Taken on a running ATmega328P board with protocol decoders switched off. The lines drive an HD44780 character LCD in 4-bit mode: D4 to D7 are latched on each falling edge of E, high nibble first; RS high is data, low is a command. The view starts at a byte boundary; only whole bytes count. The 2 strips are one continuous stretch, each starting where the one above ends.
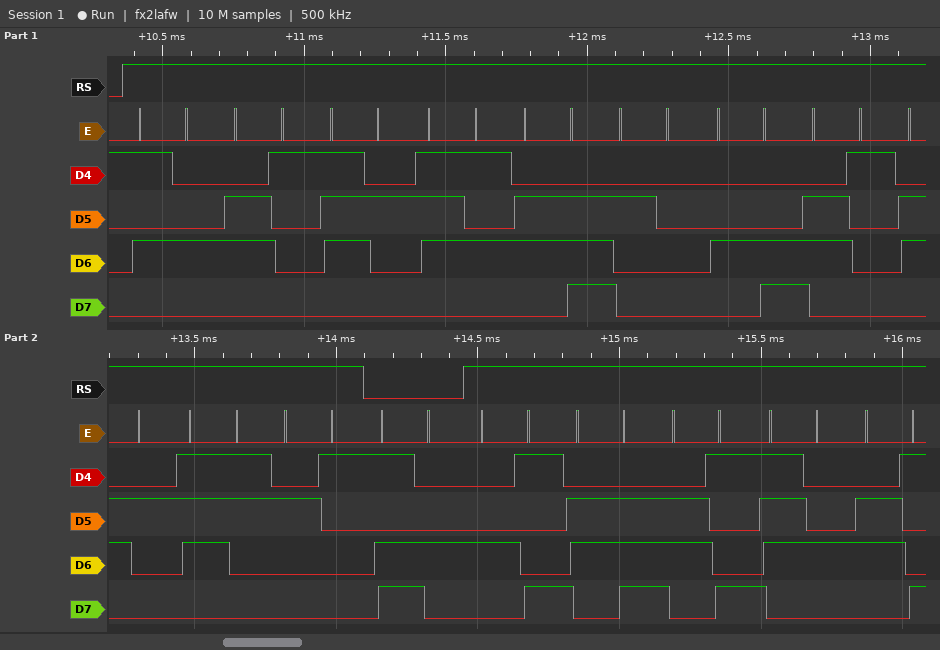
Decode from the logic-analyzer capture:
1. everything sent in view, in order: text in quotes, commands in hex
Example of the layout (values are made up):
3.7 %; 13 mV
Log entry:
"Tarun Labs!" 0xD4 "Initi"
